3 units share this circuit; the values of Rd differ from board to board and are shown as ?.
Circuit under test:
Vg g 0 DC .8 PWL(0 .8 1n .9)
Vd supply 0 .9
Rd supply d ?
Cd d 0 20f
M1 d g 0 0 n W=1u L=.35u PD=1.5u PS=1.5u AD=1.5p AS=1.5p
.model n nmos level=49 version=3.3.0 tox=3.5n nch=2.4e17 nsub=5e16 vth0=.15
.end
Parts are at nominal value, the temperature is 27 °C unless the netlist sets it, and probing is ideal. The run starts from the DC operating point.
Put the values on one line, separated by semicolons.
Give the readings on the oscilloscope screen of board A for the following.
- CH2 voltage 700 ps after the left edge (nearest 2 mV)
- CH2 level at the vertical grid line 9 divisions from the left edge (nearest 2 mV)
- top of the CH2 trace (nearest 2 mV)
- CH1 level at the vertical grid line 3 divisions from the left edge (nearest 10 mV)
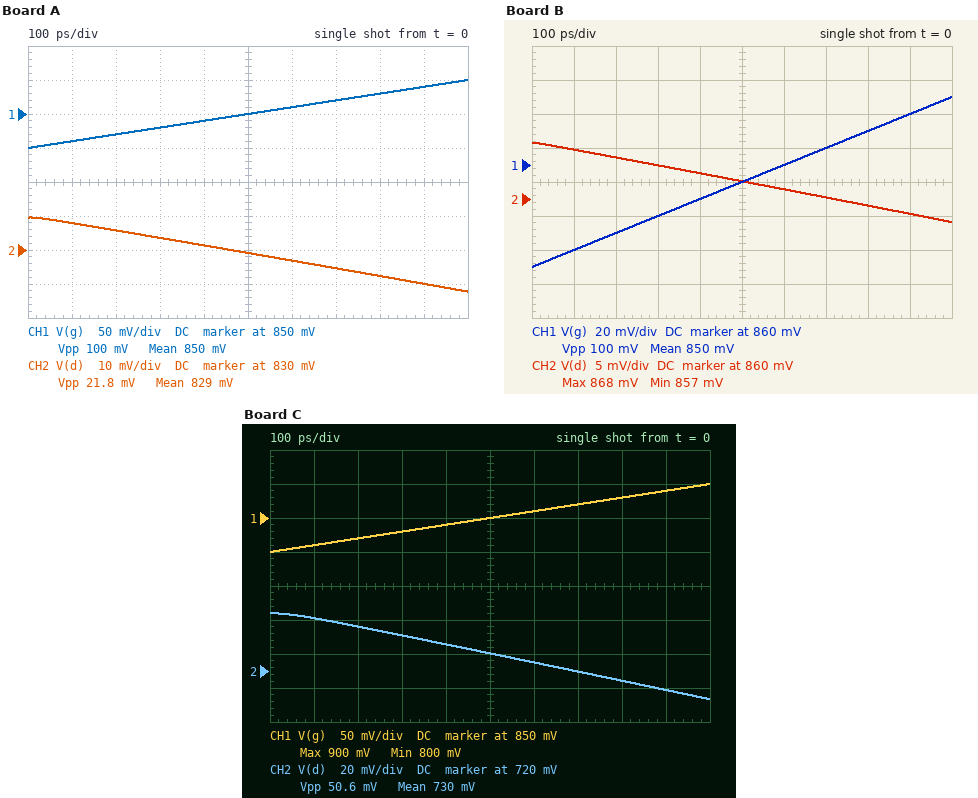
824 mV; 820 mV; 840 mV; 830 mV
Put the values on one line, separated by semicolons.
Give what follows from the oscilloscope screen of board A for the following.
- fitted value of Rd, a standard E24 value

820 Ω
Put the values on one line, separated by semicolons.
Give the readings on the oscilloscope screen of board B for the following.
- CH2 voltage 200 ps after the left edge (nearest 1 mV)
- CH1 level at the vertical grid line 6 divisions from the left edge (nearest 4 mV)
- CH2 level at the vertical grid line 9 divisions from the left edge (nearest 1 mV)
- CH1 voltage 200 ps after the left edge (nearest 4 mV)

866 mV; 860 mV; 858 mV; 820 mV
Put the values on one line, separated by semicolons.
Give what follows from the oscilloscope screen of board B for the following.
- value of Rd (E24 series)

430 Ω
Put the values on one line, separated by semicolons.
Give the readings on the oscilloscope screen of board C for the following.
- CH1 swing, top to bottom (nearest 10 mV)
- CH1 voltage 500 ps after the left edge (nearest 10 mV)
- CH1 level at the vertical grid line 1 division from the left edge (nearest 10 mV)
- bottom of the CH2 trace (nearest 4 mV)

100 mV; 850 mV; 810 mV; 704 mV
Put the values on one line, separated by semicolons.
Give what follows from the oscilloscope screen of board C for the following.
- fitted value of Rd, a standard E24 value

2 kΩ
